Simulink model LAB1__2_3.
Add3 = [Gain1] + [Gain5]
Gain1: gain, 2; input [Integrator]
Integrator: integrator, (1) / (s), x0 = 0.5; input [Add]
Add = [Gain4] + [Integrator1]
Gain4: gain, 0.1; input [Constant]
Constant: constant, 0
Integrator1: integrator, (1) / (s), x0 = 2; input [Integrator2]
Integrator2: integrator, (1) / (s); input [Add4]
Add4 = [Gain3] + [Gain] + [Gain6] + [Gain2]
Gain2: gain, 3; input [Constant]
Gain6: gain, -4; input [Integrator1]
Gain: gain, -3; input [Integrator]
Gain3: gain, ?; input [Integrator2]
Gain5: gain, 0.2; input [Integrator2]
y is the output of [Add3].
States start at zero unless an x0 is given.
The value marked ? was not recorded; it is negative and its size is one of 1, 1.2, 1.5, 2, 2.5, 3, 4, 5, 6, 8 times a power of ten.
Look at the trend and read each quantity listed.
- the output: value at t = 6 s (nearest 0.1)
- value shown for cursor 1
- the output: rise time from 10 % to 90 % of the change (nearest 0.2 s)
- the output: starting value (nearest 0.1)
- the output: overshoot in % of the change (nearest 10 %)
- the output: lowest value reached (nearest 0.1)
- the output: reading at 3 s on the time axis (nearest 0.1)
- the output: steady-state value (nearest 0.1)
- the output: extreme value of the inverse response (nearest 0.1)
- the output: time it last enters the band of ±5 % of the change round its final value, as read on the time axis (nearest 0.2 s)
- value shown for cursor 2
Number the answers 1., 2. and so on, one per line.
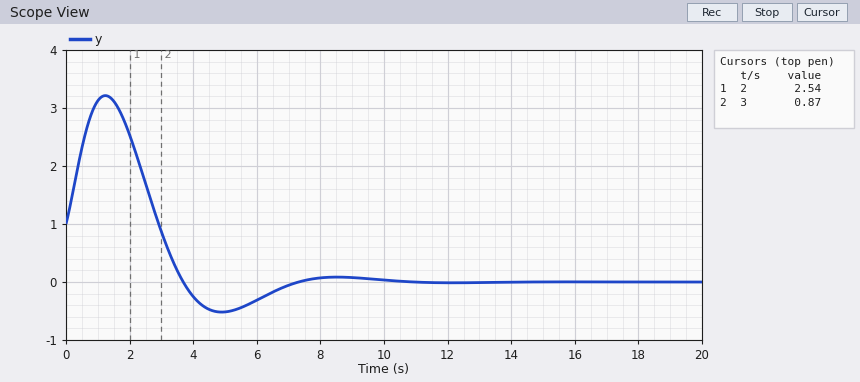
1. -0.3
2. 2.54
3. 0.6 s
4. 1.0
5. 50 %
6. -0.5
7. 0.9
8. 0.0
9. 3.2
10. 9.6 s
11. 0.87
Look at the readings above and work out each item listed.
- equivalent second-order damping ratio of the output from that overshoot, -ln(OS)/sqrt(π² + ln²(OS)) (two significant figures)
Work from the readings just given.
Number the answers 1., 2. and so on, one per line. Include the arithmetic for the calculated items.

1. ln(0.5) = -0.693; 0.693 / sqrt(9.870 + 0.480) = 0.22
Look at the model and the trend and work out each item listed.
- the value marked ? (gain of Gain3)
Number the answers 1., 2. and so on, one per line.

1. -4
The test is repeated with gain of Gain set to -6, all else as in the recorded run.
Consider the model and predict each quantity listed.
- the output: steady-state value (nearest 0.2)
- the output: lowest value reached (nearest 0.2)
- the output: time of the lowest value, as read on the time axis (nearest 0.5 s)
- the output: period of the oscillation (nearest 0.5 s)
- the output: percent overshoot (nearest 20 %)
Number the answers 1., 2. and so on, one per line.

1. 0.0
2. -1.2
3. 3.5 s
4. 5.0 s
5. 120 %
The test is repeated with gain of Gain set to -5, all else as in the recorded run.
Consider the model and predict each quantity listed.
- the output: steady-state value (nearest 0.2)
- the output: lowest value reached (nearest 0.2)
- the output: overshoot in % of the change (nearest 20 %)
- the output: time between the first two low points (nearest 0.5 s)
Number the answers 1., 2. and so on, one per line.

1. 0.0
2. -1.0
3. 100 %
4. 5.5 s
